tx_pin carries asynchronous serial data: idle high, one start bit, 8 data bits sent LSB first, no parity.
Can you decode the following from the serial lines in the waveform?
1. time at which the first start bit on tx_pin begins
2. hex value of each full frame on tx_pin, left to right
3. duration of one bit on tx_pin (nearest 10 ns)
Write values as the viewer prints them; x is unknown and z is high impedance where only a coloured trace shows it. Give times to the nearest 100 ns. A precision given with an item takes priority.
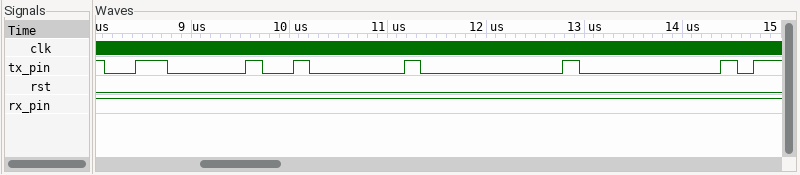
8100 ns
06, 02, 00, 00
160 ns
